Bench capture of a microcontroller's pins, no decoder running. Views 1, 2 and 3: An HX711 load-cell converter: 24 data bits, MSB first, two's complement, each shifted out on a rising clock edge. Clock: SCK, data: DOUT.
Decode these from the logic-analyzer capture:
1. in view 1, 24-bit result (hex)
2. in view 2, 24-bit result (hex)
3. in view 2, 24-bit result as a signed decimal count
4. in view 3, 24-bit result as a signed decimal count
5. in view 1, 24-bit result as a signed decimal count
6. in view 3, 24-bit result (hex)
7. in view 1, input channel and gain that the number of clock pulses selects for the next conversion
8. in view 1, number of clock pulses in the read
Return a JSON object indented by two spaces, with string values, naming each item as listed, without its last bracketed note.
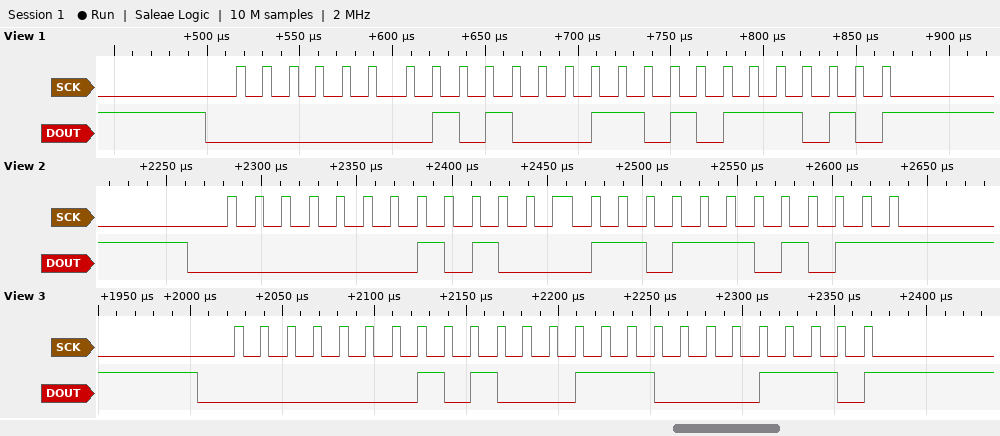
{
  "in view 1, 24-bit result": "0x0146BA",
  "in view 2, 24-bit result": "0x0146EB",
  "in view 2, 24-bit result as a signed decimal count": "83691",
  "in view 3, 24-bit result as a signed decimal count": "83726",
  "in view 1, 24-bit result as a signed decimal count": "83642",
  "in view 3, 24-bit result": "0x01470E",
  "in view 1, input channel and gain that the number of clock pulses selects for the next conversion": "channel A, gain 128",
  "in view 1, number of clock pulses in the read": "25"
}
